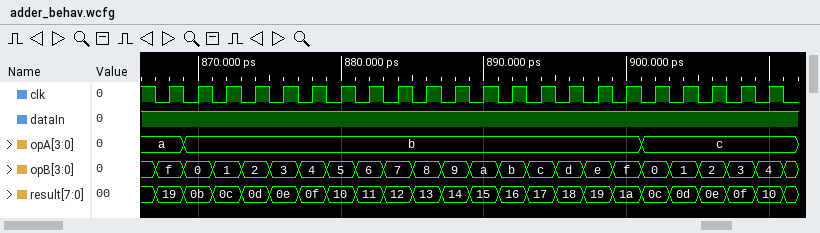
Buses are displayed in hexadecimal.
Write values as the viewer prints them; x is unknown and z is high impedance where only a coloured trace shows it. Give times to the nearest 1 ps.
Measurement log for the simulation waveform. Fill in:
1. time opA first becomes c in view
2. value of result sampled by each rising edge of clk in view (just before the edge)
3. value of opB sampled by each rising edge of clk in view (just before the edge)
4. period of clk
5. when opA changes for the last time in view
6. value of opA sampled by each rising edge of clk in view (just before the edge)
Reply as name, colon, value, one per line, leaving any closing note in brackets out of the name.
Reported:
time opA first becomes c in view: 901 ps
value of result sampled by each rising edge of clk in view: 19, 0b, 0c, 0d, 0e, 0f, 10, 11, 12, 13, 14, 15, 16, 17, 18, 19, 1a, 0c, 0d, 0e, 0f, 10
value of opB sampled by each rising edge of clk in view: f, 0, 1, 2, 3, 4, 5, 6, 7, 8, 9, a, b, c, d, e, f, 0, 1, 2, 3, 4
period of clk: 2 ps
when opA changes for the last time in view: 901 ps
value of opA sampled by each rising edge of clk in view: a, b, b, b, b, b, b, b, b, b, b, b, b, b, b, b, b, c, c, c, c, c
